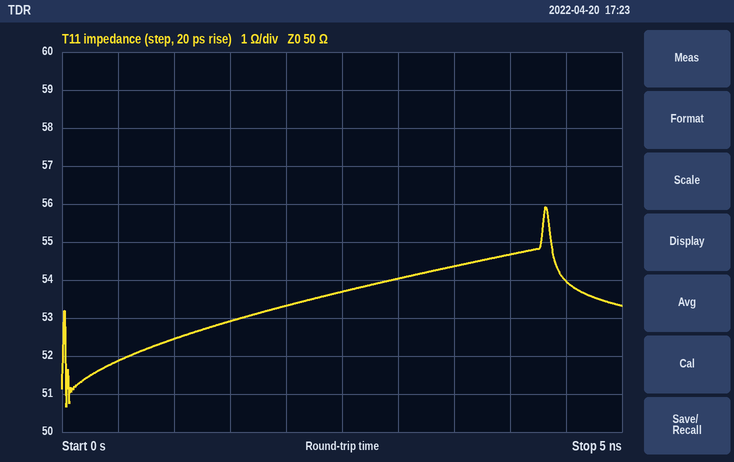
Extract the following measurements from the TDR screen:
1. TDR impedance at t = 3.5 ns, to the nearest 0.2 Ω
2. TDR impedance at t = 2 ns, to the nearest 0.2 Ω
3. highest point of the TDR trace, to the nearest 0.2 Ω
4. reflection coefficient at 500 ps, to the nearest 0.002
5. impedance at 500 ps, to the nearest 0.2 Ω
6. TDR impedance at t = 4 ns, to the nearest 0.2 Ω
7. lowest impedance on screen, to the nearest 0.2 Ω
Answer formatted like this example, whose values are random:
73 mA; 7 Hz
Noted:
54.4 Ω; 53.4 Ω; 56.0 Ω; +0.018; 51.8 Ω; 54.6 Ω; 50.6 Ω
